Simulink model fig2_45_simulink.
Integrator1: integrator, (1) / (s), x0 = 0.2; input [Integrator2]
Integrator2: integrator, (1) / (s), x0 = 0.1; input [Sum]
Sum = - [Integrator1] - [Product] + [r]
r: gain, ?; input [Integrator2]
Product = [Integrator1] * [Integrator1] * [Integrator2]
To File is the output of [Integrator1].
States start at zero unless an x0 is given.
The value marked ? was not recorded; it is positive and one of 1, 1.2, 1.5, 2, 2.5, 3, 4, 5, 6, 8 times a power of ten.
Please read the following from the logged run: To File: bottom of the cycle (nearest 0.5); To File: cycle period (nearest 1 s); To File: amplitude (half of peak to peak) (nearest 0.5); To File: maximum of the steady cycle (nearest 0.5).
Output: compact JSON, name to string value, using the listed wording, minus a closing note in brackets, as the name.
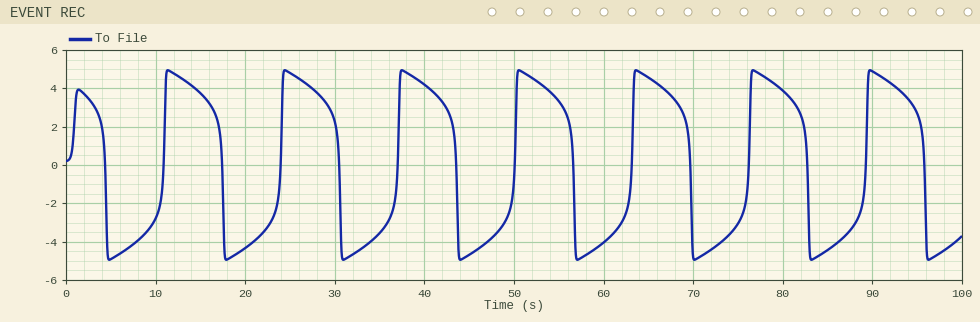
{"To File: bottom of the cycle": "-5.0", "To File: cycle period": "13 s", "To File: amplitude (half of peak to peak)": "5.0", "To File: maximum of the steady cycle": "5.0"}
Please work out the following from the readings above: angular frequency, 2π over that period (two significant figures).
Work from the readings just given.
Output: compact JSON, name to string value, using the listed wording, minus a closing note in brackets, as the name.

{"angular frequency, 2π over that period": "0.48 rad/s"}
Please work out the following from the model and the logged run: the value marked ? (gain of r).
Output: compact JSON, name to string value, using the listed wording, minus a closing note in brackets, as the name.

{"the value marked ?": "6"}
